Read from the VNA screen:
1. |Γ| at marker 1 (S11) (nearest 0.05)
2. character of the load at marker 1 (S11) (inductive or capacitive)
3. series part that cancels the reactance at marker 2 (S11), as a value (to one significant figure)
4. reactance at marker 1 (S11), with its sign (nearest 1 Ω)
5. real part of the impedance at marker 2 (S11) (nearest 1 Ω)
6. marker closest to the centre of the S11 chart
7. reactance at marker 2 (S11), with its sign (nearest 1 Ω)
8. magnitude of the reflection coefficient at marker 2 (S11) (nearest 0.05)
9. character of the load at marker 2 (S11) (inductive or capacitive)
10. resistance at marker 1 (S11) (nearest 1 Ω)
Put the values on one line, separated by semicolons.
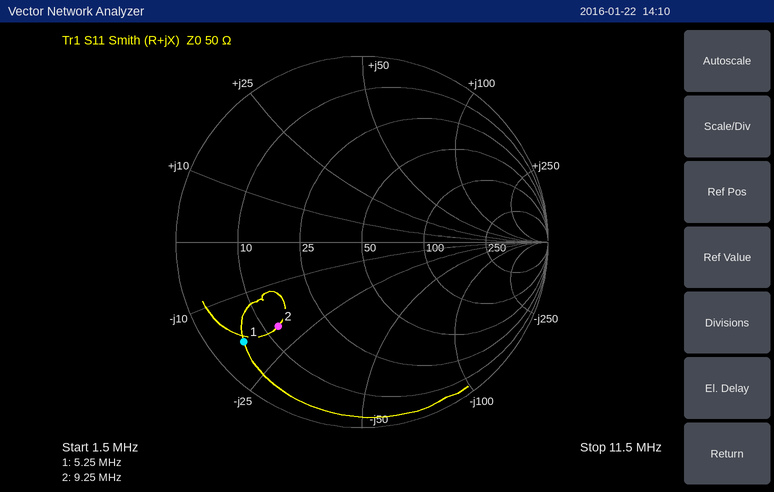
0.85; capacitive; 300 nH; -18 Ω; 13 Ω; marker 2; -20 Ω; 0.65; capacitive; 5 Ω
